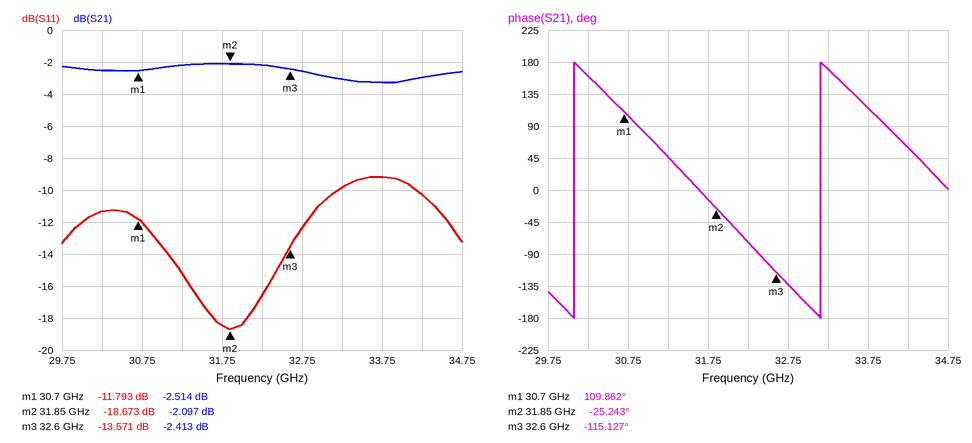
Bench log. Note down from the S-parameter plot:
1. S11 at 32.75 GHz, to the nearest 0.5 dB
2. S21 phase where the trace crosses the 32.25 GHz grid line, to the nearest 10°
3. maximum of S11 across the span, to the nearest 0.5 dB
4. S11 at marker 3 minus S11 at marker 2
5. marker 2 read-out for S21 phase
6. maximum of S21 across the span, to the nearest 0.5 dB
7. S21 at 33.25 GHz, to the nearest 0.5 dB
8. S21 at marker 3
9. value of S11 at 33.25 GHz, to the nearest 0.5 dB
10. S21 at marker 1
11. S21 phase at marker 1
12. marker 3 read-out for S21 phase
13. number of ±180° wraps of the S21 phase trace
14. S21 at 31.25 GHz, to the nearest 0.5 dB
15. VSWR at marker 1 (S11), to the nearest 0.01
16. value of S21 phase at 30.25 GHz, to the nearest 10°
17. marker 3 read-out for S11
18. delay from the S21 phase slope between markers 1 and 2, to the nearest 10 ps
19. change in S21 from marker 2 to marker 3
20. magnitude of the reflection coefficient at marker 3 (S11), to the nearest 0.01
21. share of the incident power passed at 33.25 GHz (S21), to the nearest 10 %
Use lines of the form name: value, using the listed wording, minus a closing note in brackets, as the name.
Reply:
S11 at 32.75 GHz, to the nearest 0.5 dB: -12.5 dB
S21 phase where the trace crosses the 32.25 GHz grid line, to the nearest 10°: -70°
maximum of S11 across the span, to the nearest 0.5 dB: -9.0 dB
S11 at marker 3 minus S11 at marker 2: 5.102 dB
marker 2 read-out for S21 phase: -25.243°
maximum of S21 across the span, to the nearest 0.5 dB: -2.0 dB
S21 at 33.25 GHz, to the nearest 0.5 dB: -3.0 dB
S21 at marker 3: -2.413 dB
value of S11 at 33.25 GHz, to the nearest 0.5 dB: -10.0 dB
S21 at marker 1: -2.514 dB
S21 phase at marker 1: 109.862°
marker 3 read-out for S21 phase: -115.127°
number of ±180° wraps of the S21 phase trace: 2
S21 at 31.25 GHz, to the nearest 0.5 dB: -2.0 dB
VSWR at marker 1 (S11), to the nearest 0.01: 1.69
value of S21 phase at 30.25 GHz, to the nearest 10°: 160°
marker 3 read-out for S11: -13.571 dB
delay from the S21 phase slope between markers 1 and 2, to the nearest 10 ps: 330 ps
change in S21 from marker 2 to marker 3: -0.316 dB
magnitude of the reflection coefficient at marker 3 (S11), to the nearest 0.01: 0.21
share of the incident power passed at 33.25 GHz (S21), to the nearest 10 %: 50 %
